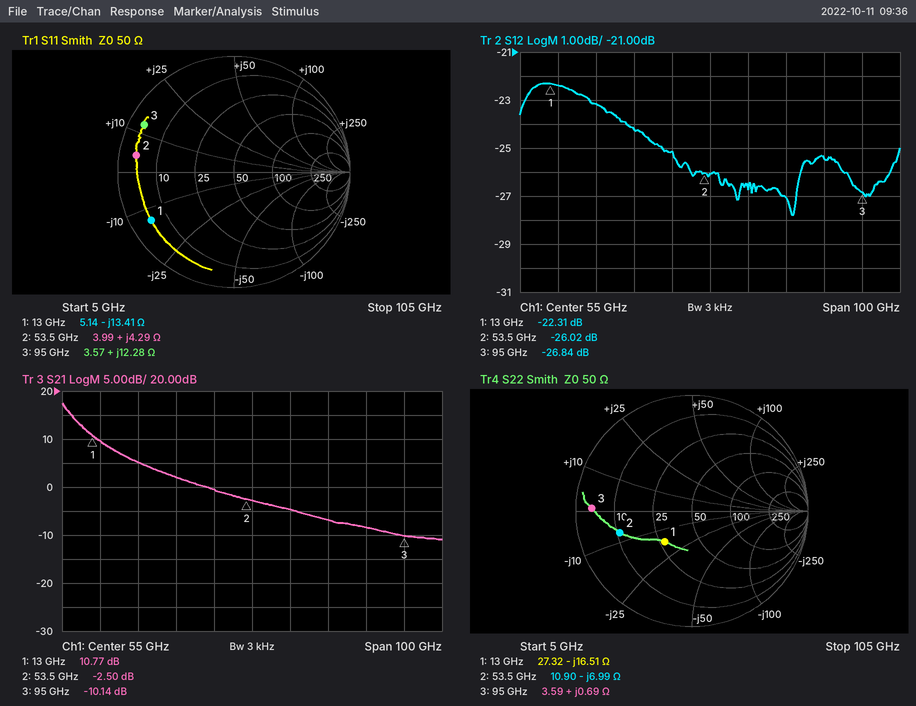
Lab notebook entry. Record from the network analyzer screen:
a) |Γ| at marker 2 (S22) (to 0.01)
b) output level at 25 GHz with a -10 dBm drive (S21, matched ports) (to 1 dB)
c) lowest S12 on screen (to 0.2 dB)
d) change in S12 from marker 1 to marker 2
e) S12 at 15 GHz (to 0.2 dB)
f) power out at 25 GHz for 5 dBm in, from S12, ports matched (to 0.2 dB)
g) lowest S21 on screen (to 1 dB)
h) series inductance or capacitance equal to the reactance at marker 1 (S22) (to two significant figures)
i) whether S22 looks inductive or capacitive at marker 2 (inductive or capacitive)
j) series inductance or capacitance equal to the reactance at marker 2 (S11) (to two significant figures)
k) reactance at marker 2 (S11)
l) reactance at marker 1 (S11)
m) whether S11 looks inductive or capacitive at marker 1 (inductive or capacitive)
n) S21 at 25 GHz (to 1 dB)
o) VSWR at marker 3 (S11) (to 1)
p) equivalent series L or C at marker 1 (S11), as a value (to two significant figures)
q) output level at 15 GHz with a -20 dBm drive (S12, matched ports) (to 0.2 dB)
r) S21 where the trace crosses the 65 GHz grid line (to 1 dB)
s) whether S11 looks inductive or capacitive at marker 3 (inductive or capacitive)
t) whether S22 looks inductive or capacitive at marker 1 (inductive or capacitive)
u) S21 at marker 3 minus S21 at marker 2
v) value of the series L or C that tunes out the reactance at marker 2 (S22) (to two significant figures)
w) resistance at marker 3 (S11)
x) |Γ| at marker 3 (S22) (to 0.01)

0.65
-5 dBm
-27.8 dB
-3.71 dB
-22.4 dB
-18.2 dBm
-11 dB
740 fF
capacitive
13 pH
+4.29 Ω
-13.41 Ω
capacitive
5 dB
15
910 fF
-42.4 dBm
-5 dB
inductive
capacitive
-7.64 dB
21 pH
3.57 Ω
0.87
